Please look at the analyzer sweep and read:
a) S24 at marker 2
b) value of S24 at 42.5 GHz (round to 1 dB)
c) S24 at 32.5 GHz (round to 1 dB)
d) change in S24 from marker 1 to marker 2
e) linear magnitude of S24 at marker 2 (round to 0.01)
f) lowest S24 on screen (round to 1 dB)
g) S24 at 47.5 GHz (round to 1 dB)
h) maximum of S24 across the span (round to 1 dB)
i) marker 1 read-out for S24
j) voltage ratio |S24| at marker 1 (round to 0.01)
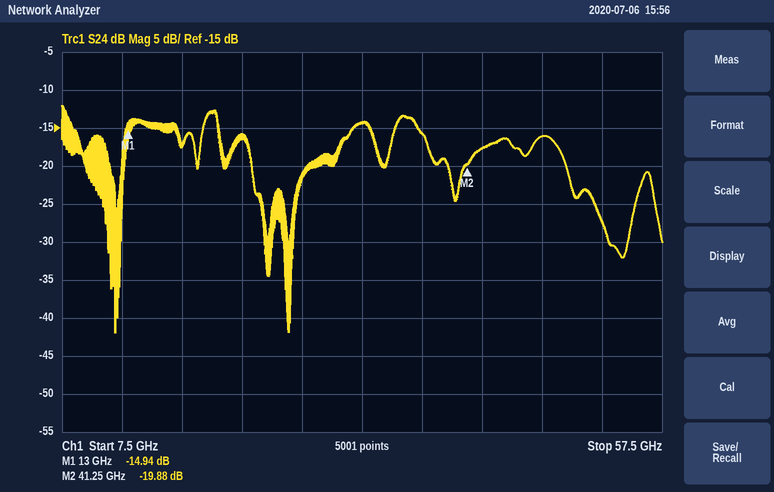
-19.88 dB
-18 dB
-14 dB
-4.94 dB
0.10
-42 dB
-16 dB
-12 dB
-14.94 dB
0.18
